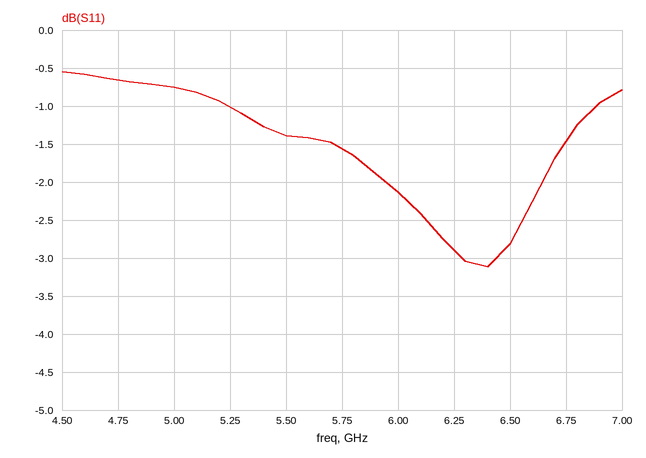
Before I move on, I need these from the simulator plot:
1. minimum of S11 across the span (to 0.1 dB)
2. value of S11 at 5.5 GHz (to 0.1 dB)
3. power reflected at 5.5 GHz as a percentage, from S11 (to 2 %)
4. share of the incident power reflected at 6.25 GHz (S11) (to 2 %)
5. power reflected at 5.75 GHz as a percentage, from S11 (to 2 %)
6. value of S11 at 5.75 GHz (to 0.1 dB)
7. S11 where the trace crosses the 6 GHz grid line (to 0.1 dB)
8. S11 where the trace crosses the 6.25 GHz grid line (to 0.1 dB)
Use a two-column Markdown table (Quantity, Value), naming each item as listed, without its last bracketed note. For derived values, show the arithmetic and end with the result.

| Quantity | Value |
|---|---|
| minimum of S11 across the span | -3.1 dB |
| value of S11 at 5.5 GHz | -1.4 dB |
| power reflected at 5.5 GHz as a percentage, from S11 | 10^(-1.4/10) ≈ 72 % |
| share of the incident power reflected at 6.25 GHz (S11) | 10^(-2.9/10) ≈ 51.3 %, so 52 % to the nearest 2 % |
| power reflected at 5.75 GHz as a percentage, from S11 | 10^(-1.6/10) ≈ 69.2 %, so 70 % to the nearest 2 % |
| value of S11 at 5.75 GHz | -1.6 dB |
| S11 where the trace crosses the 6 GHz grid line | -2.1 dB |
| S11 where the trace crosses the 6.25 GHz grid line | -2.9 dB |
